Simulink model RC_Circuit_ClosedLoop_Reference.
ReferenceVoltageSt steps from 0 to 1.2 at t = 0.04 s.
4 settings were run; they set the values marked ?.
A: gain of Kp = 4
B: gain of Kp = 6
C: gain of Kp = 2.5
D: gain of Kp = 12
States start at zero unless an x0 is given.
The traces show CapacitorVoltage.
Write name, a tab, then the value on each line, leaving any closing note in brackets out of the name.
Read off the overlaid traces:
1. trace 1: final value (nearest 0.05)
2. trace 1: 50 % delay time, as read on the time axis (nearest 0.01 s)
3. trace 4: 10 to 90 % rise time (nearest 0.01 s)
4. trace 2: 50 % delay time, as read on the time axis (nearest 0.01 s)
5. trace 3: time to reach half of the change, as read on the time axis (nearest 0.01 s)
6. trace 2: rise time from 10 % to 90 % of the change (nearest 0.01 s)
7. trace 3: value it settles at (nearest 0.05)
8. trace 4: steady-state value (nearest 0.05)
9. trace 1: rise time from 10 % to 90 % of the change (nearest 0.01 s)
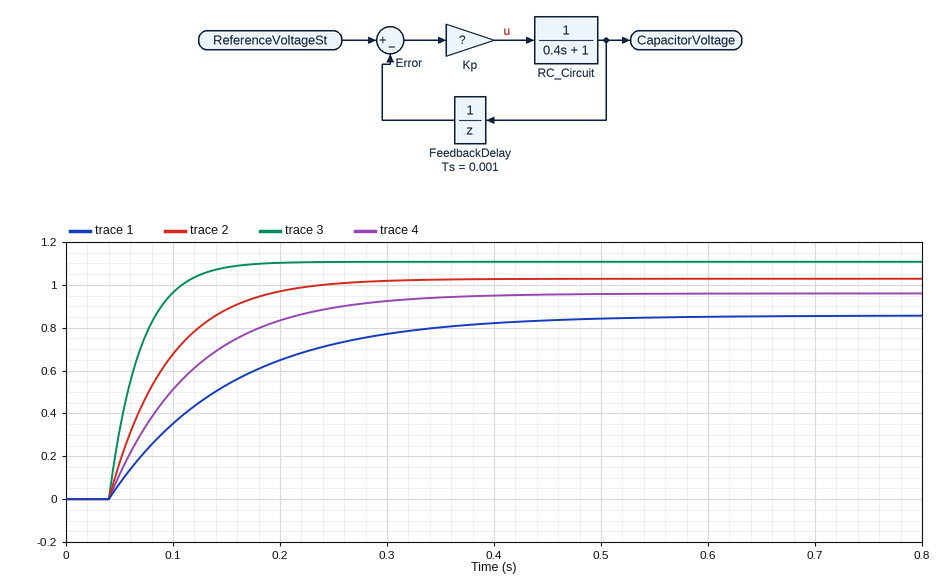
trace 1: final value	0.85
trace 1: 50 % delay time, as read on the time axis	0.12 s
trace 4: 10 to 90 % rise time	0.17 s
trace 2: 50 % delay time, as read on the time axis	0.08 s
trace 3: time to reach half of the change, as read on the time axis	0.06 s
trace 2: rise time from 10 % to 90 % of the change	0.12 s
trace 3: value it settles at	1.10
trace 4: steady-state value	0.95
trace 1: rise time from 10 % to 90 % of the change	0.25 s
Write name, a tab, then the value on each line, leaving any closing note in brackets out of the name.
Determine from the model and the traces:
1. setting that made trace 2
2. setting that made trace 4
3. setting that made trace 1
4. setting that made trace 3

setting that made trace 2	B
setting that made trace 4	A
setting that made trace 1	C
setting that made trace 3	D
